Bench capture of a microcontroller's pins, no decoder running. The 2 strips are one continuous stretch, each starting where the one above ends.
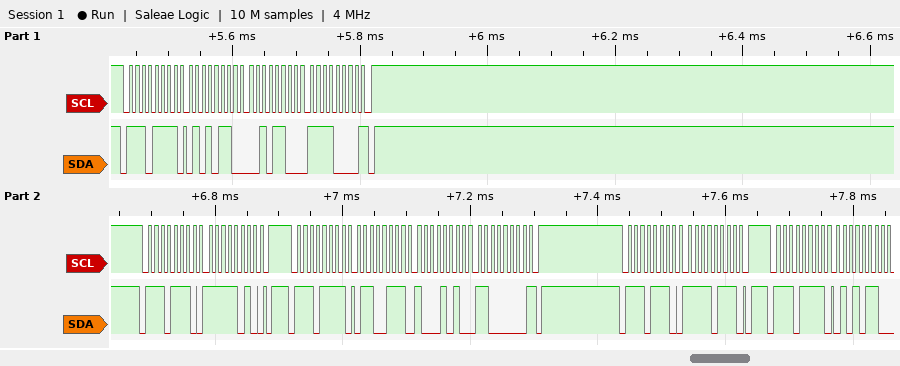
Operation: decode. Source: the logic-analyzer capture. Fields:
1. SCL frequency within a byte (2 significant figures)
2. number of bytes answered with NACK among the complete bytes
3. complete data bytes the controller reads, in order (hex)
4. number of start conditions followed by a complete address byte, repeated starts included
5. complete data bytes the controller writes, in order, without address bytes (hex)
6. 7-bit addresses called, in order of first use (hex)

100 kHz
2
56 2C F0 67 8A C0 56
5
FA F7
0x77
